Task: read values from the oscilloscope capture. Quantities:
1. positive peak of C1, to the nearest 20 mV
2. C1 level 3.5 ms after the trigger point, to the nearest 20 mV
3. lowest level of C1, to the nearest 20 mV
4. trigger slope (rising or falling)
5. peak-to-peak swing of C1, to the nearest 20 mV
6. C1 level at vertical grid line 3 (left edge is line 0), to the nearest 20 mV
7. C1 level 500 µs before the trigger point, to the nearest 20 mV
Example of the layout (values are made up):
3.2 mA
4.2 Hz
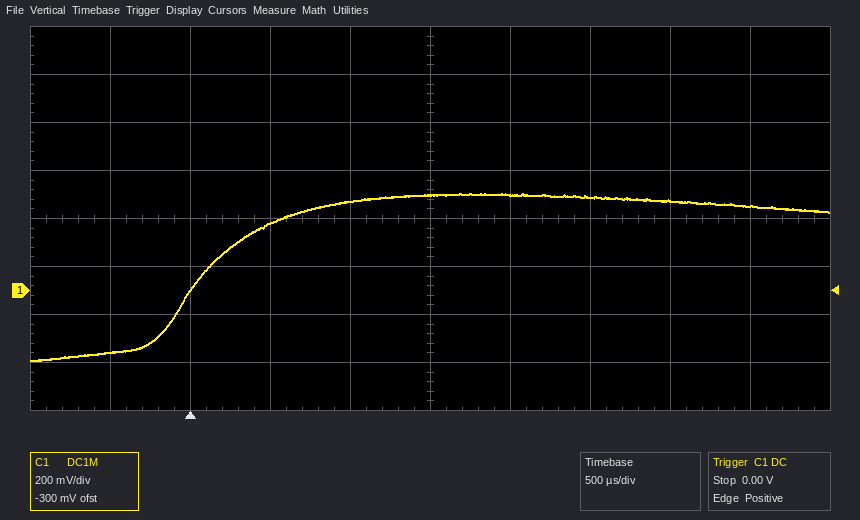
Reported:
400 mV
360 mV
-300 mV
rising
700 mV
280 mV
-260 mV
